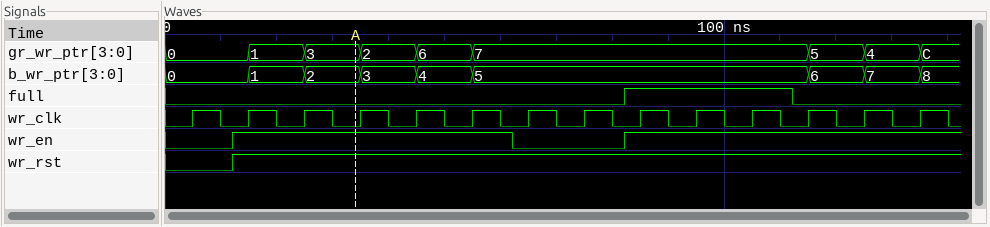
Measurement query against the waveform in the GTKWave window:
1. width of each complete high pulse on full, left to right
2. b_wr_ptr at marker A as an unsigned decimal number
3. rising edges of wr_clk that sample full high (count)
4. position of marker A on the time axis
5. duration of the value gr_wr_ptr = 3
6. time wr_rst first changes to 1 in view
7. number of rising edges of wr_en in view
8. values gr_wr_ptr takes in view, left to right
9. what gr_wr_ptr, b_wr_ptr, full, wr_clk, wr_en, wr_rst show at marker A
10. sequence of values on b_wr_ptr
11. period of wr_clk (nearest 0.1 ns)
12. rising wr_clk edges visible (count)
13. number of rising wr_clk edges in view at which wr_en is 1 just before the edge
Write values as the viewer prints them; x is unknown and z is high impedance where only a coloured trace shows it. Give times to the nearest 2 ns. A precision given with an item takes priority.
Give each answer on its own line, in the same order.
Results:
30 ns
2
3
34 ns
10 ns
12 ns
2
0, 1, 3, 2, 6, 7, 5, 4, C
gr_wr_ptr=3, b_wr_ptr=2, full=0, wr_clk=0, wr_en=1, wr_rst=1
0, 1, 2, 3, 4, 5, 6, 7, 8
10 ns
14
11
